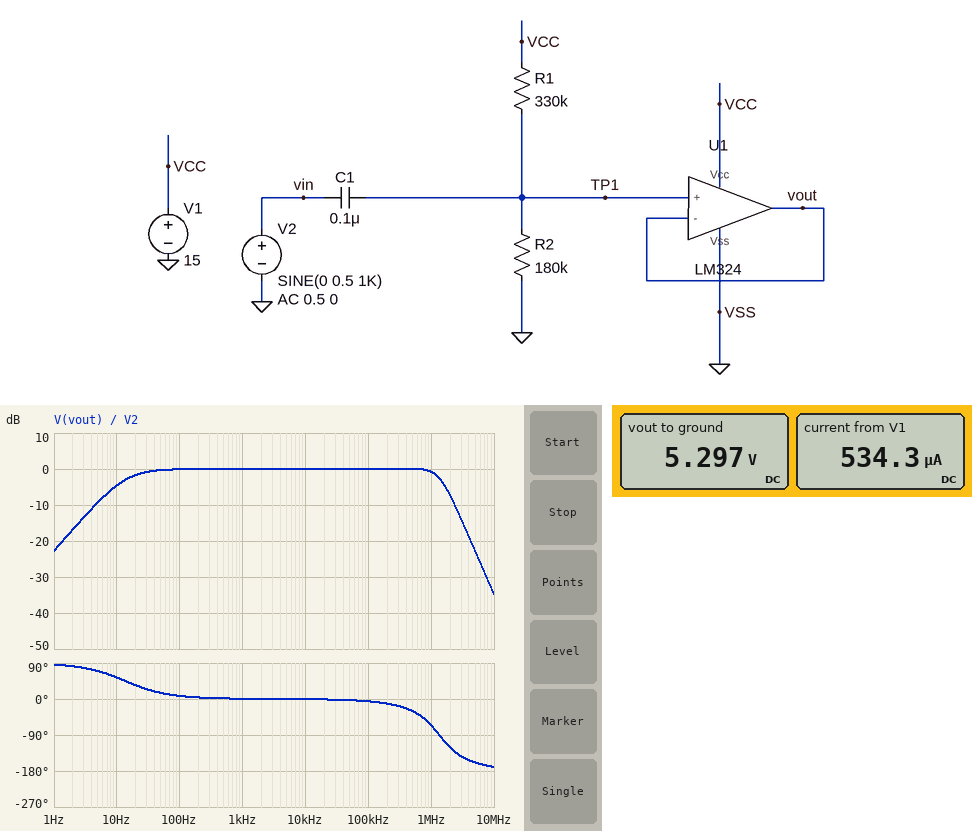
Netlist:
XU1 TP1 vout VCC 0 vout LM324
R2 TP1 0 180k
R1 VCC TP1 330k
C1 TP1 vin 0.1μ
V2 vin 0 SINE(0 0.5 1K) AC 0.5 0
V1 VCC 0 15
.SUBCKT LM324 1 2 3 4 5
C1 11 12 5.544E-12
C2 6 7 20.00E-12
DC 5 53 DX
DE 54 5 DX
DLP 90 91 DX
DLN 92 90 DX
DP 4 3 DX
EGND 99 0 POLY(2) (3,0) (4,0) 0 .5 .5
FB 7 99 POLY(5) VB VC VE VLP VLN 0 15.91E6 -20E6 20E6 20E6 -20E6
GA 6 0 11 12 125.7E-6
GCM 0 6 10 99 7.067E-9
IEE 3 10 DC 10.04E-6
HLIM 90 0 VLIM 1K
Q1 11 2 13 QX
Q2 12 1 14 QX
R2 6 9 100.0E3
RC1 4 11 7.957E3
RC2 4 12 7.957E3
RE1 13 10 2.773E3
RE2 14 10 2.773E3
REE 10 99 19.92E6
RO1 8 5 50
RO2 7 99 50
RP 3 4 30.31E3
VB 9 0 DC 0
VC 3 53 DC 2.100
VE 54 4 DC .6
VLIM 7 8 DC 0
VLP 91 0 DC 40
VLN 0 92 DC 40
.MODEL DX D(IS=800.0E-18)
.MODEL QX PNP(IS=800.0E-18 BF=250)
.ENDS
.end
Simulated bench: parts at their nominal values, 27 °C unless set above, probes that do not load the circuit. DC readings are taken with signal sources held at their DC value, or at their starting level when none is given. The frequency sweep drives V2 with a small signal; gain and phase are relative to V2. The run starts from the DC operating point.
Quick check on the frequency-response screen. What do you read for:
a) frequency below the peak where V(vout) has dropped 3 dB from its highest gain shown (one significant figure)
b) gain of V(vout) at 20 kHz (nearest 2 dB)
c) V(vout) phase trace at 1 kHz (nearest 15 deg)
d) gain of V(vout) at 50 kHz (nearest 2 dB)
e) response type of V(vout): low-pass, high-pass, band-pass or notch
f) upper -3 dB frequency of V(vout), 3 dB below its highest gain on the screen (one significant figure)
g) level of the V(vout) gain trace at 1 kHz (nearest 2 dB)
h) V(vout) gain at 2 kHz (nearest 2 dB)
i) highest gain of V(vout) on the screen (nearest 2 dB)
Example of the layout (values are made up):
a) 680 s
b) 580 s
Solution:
a) 10 Hz
b) 0 dB
c) 0 deg
d) 0 dB
e) band-pass
f) 1 MHz
g) 0 dB
h) 0 dB
i) 0 dB
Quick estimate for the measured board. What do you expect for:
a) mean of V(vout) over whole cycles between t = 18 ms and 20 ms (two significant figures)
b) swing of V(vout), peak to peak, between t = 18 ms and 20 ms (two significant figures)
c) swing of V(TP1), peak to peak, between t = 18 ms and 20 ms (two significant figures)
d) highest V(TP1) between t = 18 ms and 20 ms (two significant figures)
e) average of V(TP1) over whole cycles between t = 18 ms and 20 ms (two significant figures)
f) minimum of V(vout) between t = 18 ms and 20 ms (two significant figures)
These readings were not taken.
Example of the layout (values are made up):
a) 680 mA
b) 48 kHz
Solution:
a) 5.3 V
b) 1.0 V
c) 1.0 V
d) 5.8 V
e) 5.3 V
f) 4.8 V
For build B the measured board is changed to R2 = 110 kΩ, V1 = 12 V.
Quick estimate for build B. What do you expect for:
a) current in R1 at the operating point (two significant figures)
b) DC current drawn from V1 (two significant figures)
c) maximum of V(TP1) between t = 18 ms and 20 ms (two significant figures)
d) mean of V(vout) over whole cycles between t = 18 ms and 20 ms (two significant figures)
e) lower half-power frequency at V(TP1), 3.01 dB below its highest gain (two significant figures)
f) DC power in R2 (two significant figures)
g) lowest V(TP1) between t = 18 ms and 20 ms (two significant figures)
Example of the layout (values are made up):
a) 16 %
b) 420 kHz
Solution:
a) 27 µA
b) 430 µA
c) 3.5 V
d) 3.0 V
e) 19 Hz
f) 82 µW
g) 2.5 V
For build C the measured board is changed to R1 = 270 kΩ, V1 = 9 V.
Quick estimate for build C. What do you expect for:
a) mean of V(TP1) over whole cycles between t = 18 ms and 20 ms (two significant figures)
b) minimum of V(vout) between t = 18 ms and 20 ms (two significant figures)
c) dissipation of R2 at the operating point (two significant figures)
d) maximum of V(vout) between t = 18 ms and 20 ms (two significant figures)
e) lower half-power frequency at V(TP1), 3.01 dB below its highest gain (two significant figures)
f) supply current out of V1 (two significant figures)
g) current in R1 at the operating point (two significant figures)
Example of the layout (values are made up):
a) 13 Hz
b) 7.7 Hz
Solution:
a) 3.6 V
b) 3.1 V
c) 72 µW
d) 4.1 V
e) 15 Hz
f) 330 µA
g) 20 µA
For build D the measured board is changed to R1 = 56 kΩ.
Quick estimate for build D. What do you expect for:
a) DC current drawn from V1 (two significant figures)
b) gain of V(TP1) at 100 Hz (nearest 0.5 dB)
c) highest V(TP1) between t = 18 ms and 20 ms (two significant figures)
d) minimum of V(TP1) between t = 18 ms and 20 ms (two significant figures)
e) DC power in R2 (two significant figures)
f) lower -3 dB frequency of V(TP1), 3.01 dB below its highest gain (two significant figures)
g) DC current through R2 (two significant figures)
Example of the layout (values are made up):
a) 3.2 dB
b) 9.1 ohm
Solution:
a) 570 µA
b) -0.5 dB
c) 12 V
d) 11 V
e) 730 µW
f) 37 Hz
g) 64 µA
